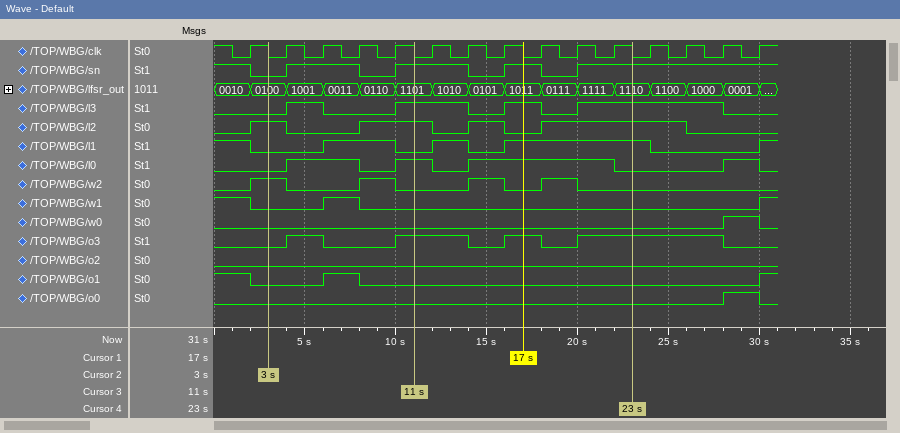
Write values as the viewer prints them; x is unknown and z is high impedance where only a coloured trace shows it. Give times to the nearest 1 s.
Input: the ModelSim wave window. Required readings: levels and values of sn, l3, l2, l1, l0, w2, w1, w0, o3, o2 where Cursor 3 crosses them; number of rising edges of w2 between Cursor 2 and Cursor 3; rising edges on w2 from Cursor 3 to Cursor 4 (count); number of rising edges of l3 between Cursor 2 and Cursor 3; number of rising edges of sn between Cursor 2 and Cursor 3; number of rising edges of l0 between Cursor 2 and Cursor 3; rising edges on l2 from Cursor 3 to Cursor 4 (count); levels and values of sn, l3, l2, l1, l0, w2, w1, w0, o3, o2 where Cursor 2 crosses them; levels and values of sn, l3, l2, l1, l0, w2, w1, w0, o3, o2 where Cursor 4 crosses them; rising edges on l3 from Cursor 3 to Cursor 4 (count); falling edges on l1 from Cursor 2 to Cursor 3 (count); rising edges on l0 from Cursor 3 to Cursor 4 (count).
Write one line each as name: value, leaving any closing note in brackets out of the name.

levels and values of sn, l3, l2, l1, l0, w2, w1, w0, o3, o2 where Cursor 3 crosses them: sn=1, l3=1, l2=1, l1=0, l0=1, w2=0, w1=0, w0=0, o3=1, o2=0
number of rising edges of w2 between Cursor 2 and Cursor 3: 1
rising edges on w2 from Cursor 3 to Cursor 4: 2
number of rising edges of l3 between Cursor 2 and Cursor 3: 2
number of rising edges of sn between Cursor 2 and Cursor 3: 2
number of rising edges of l0 between Cursor 2 and Cursor 3: 2
rising edges on l2 from Cursor 3 to Cursor 4: 2
levels and values of sn, l3, l2, l1, l0, w2, w1, w0, o3, o2 where Cursor 2 crosses them: sn=0, l3=0, l2=1, l1=0, l0=0, w2=1, w1=0, w0=0, o3=0, o2=0
levels and values of sn, l3, l2, l1, l0, w2, w1, w0, o3, o2 where Cursor 4 crosses them: sn=1, l3=1, l2=1, l1=1, l0=0, w2=0, w1=0, w0=0, o3=1, o2=0
rising edges on l3 from Cursor 3 to Cursor 4: 2
falling edges on l1 from Cursor 2 to Cursor 3: 1
rising edges on l0 from Cursor 3 to Cursor 4: 1
